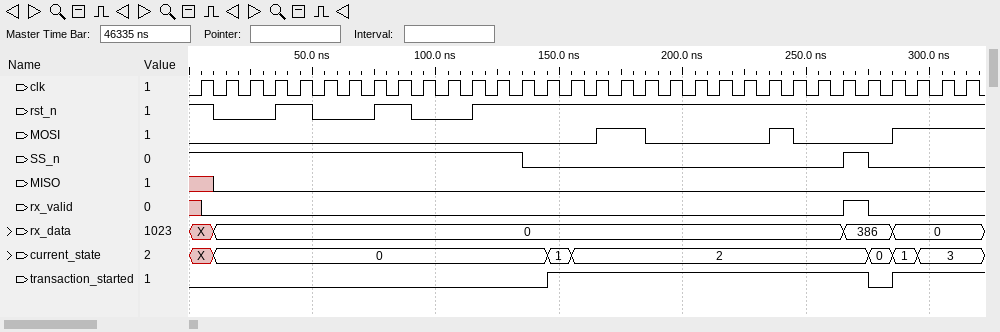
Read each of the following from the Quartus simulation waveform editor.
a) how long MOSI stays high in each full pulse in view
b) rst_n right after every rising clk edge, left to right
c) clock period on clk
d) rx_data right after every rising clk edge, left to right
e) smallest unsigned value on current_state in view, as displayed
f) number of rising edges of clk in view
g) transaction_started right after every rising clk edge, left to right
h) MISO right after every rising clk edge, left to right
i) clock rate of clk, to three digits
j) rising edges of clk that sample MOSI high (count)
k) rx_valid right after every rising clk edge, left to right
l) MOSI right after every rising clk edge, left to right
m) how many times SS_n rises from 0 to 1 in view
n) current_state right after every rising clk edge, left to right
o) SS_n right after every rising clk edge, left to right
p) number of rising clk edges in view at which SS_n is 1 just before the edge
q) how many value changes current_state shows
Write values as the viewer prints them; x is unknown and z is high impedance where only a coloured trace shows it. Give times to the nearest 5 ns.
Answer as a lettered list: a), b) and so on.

a) 20 ns, 10 ns
b) 1 0 0 1 1 0 0 1 1 0 0 1 1 1 1 1 1 1 1 1 1 1 1 1 1 1 1 1 1 1 1 1
c) 10 ns
d) X, 0, 0, 0, 0, 0, 0, 0, 0, 0, 0, 0, 0, 0, 0, 0, 0, 0, 0, 0, 0, 0, 0, 0, 0, 0, 386, 386, 0, 0, 0, 0
e) 0
f) 32
g) 0 0 0 0 0 0 0 0 0 0 0 0 0 0 1 1 1 1 1 1 1 1 1 1 1 1 1 0 1 1 1 1
h) x 0 0 0 0 0 0 0 0 0 0 0 0 0 0 0 0 0 0 0 0 0 0 0 0 0 0 0 0 0 0 0
i) 100 MHz
j) 6
k) 0 0 0 0 0 0 0 0 0 0 0 0 0 0 0 0 0 0 0 0 0 0 0 0 0 0 1 0 0 0 0 0
l) 0 0 0 0 0 0 0 0 0 0 0 0 0 0 0 0 1 1 0 0 0 0 0 1 0 0 0 0 1 1 1 1
m) 1
n) X, 0, 0, 0, 0, 0, 0, 0, 0, 0, 0, 0, 0, 0, 1, 2, 2, 2, 2, 2, 2, 2, 2, 2, 2, 2, 2, 0, 1, 3, 3, 3
o) 1 1 1 1 1 1 1 1 1 1 1 1 1 0 0 0 0 0 0 0 0 0 0 0 0 0 1 0 0 0 0 0
p) 15
q) 6
